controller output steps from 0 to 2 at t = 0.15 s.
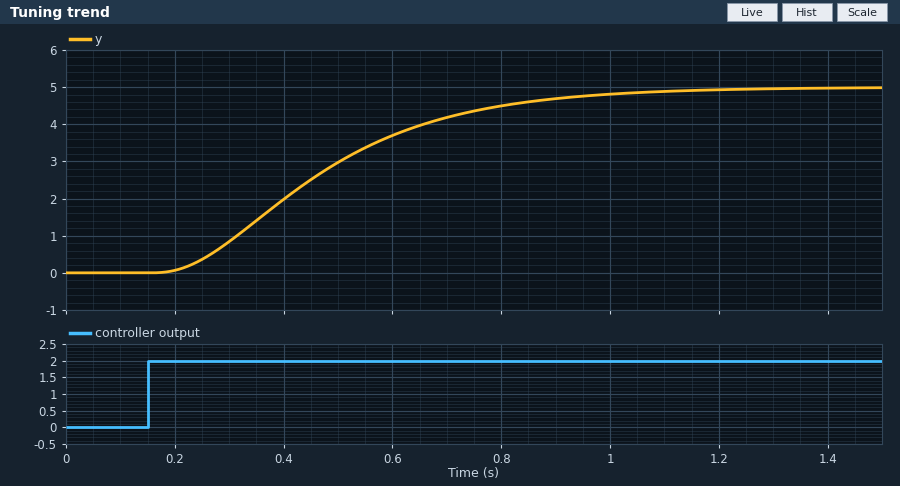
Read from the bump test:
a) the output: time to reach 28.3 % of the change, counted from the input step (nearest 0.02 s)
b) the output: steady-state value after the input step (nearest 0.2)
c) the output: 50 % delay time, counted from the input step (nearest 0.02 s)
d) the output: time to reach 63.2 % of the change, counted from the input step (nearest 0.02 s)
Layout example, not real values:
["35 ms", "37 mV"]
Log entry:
["0.20 s", "5.0", "0.30 s", "0.38 s"]
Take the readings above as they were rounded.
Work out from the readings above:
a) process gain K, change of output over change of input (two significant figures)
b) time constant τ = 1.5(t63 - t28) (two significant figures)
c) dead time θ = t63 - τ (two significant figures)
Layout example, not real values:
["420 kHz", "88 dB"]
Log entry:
["2.5", "0.27 s", "0.11 s"]
